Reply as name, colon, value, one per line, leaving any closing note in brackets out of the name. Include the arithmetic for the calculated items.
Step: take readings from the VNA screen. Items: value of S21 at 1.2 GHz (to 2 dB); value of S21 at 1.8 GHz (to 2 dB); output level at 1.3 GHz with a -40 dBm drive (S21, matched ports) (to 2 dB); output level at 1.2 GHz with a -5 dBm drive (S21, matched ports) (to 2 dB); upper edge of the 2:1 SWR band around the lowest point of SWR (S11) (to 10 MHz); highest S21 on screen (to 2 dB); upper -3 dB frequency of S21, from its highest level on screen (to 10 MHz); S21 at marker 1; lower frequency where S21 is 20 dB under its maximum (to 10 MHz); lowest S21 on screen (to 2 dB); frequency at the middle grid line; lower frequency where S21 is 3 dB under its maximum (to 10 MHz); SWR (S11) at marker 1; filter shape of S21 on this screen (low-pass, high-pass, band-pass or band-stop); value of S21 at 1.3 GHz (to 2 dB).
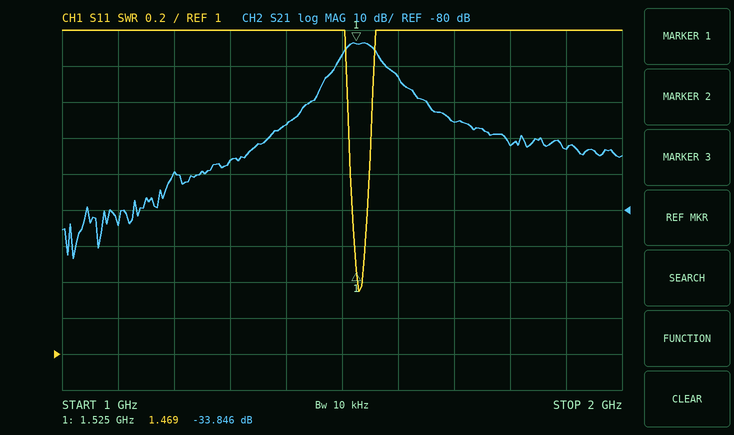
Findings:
value of S21 at 1.2 GHz: -70 dB
value of S21 at 1.8 GHz: -62 dB
output level at 1.3 GHz with a -40 dBm drive (S21, matched ports): -40 dBm + (-66 dB) = -106 dBm
output level at 1.2 GHz with a -5 dBm drive (S21, matched ports): -5 dBm + (-70 dB) = -74 dBm
upper edge of the 2:1 SWR band around the lowest point of SWR (S11): 1.55 GHz
highest S21 on screen: -34 dB
upper -3 dB frequency of S21, from its highest level on screen: 1.56 GHz
S21 at marker 1: -33.846 dB
lower frequency where S21 is 20 dB under its maximum: 1.42 GHz
lowest S21 on screen: -94 dB
frequency at the middle grid line: 1.5 GHz
lower frequency where S21 is 3 dB under its maximum: 1.50 GHz
SWR (S11) at marker 1: 1.469
filter shape of S21 on this screen: band-pass
value of S21 at 1.3 GHz: -66 dB
